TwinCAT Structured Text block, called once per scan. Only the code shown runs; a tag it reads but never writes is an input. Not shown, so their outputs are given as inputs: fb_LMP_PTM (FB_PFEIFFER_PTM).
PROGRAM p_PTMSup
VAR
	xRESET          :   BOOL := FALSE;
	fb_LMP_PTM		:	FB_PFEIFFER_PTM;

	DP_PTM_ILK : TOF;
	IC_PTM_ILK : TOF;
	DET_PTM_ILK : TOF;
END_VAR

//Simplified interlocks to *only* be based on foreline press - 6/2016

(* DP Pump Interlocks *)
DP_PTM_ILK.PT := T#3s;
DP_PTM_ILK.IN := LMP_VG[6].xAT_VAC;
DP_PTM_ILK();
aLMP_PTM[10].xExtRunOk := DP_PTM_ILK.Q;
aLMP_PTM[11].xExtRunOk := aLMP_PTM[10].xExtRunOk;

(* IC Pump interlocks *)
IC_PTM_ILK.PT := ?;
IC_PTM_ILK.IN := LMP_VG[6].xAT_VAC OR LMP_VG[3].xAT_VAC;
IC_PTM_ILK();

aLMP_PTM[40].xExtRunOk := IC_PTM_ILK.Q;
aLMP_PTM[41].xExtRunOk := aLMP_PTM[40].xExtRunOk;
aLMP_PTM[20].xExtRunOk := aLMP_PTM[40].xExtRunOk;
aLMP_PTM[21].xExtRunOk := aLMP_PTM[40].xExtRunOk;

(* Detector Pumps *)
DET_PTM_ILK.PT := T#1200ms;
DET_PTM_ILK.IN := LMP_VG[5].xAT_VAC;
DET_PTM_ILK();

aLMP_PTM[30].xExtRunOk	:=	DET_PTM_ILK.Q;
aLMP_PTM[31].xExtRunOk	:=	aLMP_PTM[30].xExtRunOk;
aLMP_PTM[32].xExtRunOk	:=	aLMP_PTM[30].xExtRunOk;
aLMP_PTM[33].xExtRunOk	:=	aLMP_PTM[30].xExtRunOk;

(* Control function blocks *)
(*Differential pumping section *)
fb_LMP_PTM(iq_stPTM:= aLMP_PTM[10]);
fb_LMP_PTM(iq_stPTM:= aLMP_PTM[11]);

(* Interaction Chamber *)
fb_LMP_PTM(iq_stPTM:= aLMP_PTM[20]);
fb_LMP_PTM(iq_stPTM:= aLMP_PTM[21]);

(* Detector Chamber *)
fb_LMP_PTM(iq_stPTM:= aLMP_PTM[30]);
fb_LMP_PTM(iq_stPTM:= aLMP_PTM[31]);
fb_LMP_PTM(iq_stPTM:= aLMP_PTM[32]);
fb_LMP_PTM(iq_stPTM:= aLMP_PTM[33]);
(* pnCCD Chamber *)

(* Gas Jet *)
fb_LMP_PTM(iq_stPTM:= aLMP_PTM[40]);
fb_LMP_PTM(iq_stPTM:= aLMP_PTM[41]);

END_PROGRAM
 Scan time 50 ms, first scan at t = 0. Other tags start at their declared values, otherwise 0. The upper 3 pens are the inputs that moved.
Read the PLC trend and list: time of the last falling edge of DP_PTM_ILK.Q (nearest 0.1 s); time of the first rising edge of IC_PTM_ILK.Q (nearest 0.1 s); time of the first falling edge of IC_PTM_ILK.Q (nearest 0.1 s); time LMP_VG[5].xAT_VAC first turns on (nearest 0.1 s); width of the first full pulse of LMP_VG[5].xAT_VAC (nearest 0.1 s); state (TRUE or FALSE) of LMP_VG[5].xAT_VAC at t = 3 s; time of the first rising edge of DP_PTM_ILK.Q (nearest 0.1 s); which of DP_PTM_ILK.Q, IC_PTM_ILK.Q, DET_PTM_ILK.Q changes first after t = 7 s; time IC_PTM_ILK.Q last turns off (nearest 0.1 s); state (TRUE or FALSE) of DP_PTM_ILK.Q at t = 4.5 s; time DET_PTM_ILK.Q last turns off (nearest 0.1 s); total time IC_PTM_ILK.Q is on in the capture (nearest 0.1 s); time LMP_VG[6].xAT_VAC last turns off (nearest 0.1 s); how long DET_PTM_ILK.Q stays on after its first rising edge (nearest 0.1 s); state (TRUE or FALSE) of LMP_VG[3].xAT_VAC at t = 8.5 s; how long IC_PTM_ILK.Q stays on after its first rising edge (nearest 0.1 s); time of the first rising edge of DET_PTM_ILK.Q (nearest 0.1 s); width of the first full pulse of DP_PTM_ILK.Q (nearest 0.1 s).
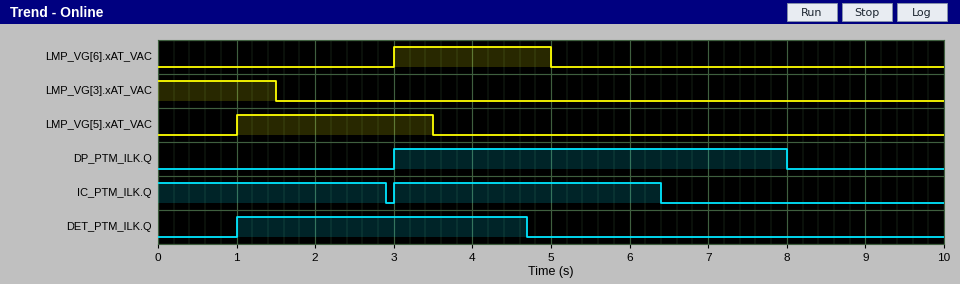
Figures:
8.0 s
3.0 s
2.9 s
1.0 s
2.5 s
TRUE
3.0 s
DP_PTM_ILK.Q
6.4 s
TRUE
4.7 s
6.3 s
5.0 s
3.7 s
FALSE
3.4 s
1.0 s
5.0 s
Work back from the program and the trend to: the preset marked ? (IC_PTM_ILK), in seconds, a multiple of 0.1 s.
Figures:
1.4 s
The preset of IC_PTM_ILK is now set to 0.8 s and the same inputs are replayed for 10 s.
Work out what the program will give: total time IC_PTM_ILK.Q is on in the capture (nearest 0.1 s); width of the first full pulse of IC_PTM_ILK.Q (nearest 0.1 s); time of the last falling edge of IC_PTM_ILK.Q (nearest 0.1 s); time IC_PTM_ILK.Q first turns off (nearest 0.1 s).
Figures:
5.1 s
2.8 s
5.8 s
2.3 s
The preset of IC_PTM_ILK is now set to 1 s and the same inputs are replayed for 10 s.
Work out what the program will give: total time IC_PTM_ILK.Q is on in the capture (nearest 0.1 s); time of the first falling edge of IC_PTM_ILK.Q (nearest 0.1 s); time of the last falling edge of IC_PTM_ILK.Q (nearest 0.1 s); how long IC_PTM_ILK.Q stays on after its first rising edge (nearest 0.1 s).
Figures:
5.5 s
2.5 s
6.0 s
3.0 s
